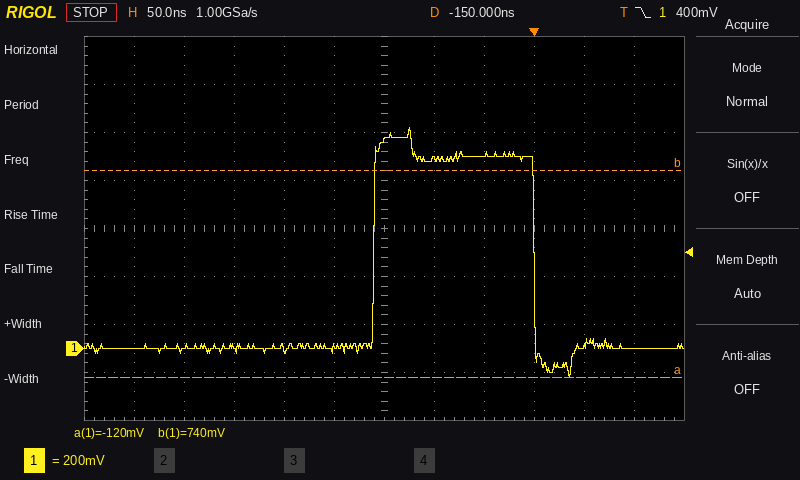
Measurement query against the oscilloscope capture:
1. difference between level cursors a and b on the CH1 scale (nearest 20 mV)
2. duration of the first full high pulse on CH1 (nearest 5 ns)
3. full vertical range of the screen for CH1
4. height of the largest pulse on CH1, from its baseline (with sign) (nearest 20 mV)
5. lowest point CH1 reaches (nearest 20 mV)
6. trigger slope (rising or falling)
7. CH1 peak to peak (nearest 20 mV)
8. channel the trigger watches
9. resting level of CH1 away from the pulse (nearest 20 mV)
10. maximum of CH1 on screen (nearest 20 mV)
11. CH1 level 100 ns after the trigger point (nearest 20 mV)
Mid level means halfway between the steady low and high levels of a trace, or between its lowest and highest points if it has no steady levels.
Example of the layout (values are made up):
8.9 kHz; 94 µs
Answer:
860 mV; 160 ns; 1.6 V; +920 mV; -120 mV; falling; 1.04 V; CH1; 0 mV; 920 mV; 0 mV
